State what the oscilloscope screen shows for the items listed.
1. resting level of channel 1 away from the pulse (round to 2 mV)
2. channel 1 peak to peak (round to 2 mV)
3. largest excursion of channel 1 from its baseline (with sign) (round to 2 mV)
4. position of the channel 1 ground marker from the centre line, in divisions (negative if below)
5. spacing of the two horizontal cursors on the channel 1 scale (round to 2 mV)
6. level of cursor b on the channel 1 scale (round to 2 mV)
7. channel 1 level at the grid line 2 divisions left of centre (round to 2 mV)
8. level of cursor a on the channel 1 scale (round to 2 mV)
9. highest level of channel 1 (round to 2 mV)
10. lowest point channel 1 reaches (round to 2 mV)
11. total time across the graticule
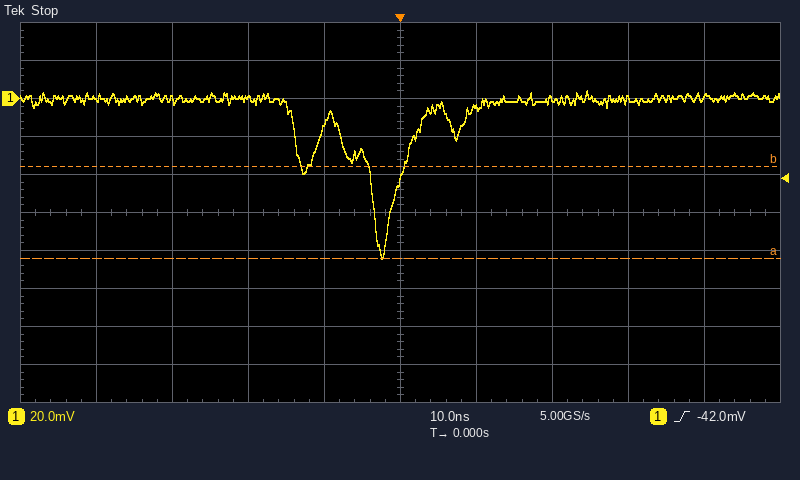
0 mV
88 mV
-84 mV
+3.0 div
48 mV
-36 mV
0 mV
-84 mV
4 mV
-84 mV
100 ns
